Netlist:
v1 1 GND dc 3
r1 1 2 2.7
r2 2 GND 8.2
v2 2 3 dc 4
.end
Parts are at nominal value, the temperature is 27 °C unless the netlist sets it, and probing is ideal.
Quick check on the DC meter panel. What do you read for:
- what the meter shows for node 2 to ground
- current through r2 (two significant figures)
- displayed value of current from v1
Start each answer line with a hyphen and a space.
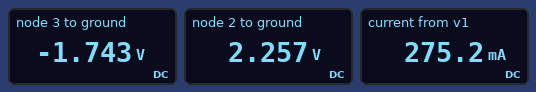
- 2.257 V
- 280 mA
- 275.2 mA
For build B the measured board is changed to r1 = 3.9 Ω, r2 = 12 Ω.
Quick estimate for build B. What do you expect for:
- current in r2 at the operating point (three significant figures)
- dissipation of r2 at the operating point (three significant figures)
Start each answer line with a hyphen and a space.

- 189 mA
- 427 mW
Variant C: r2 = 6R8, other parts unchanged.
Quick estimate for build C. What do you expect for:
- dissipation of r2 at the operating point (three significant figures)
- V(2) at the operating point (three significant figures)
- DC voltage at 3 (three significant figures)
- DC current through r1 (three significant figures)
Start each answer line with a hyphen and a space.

- 678 mW
- 2.15 V
- -1.85 V
- 316 mA
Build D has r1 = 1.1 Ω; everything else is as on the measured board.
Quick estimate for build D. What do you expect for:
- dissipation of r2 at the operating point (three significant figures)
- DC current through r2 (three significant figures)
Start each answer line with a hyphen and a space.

- 853 mW
- 323 mA
